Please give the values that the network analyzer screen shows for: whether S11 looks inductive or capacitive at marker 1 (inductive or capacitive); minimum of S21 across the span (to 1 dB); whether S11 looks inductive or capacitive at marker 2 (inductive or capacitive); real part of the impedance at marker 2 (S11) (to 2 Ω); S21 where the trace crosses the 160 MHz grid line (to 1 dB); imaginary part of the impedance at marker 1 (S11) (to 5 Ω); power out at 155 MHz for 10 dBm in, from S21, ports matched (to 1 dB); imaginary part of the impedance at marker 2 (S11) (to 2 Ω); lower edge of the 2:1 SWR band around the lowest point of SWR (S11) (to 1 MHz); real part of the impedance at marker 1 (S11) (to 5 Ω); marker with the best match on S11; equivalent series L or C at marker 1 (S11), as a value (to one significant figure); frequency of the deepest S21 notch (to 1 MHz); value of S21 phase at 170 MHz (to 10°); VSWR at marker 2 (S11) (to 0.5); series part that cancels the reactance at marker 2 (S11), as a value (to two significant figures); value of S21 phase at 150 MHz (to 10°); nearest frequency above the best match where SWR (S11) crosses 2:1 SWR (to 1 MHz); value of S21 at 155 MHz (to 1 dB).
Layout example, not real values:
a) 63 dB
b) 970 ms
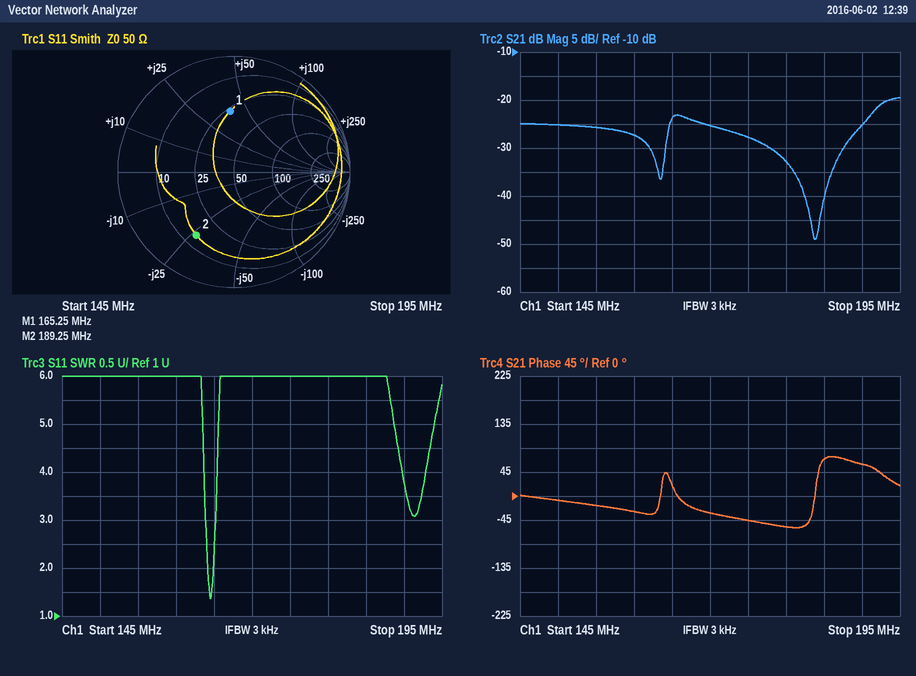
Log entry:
a) inductive
b) -49 dB
c) capacitive
d) 14 Ω
e) -27 dB
f) +40 Ω
g) -16 dBm
h) -26 Ω
i) 164 MHz
j) 25 Ω
k) marker 1
l) 40 nH
m) 184 MHz
n) -30°
o) 4.5
p) 22 nH
q) -10°
r) 165 MHz
s) -26 dB
